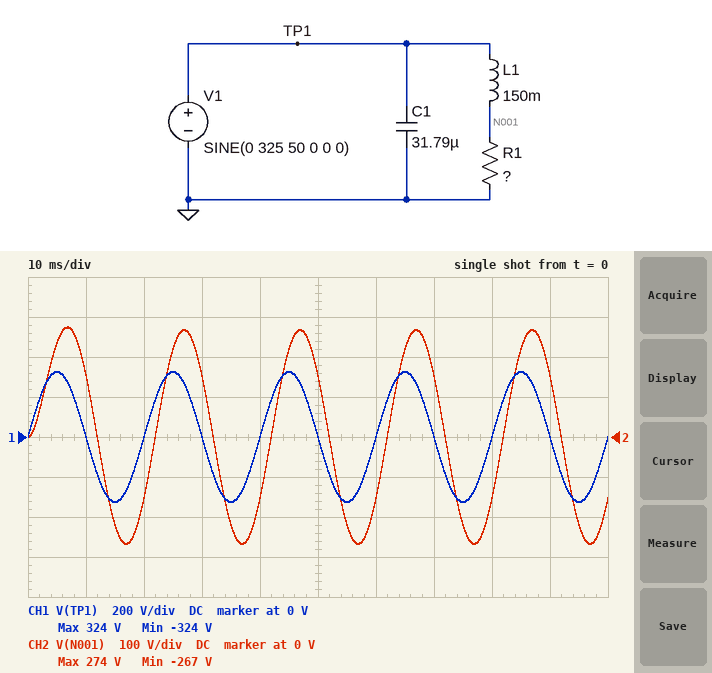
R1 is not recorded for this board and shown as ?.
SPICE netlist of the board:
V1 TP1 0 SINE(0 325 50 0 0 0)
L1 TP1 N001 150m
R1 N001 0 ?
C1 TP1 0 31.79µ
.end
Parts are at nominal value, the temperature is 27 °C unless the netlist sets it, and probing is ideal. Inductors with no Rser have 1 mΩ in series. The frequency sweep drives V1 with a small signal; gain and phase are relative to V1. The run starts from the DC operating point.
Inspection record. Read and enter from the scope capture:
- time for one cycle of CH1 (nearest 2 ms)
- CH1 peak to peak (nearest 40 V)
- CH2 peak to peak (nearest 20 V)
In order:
20 ms
640 V
540 V
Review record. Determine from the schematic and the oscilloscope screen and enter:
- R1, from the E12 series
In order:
68 Ω
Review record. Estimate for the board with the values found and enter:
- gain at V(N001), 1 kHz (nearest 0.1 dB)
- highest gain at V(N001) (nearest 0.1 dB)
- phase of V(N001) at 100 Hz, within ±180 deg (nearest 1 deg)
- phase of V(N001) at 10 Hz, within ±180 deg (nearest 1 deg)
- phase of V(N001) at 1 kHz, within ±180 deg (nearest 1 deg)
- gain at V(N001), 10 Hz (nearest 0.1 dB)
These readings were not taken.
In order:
-22.9 dB
0 dB
-54 deg
-8 deg
-86 deg
-0.1 dB
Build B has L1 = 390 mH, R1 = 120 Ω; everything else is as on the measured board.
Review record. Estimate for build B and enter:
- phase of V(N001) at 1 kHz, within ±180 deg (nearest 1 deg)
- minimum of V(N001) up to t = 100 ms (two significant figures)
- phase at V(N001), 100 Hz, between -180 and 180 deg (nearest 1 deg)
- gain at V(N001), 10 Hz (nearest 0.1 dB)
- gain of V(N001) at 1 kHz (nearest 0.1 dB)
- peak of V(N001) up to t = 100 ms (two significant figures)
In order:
-87 deg
-230 V
-64 deg
-0.2 dB
-26.2 dB
240 V
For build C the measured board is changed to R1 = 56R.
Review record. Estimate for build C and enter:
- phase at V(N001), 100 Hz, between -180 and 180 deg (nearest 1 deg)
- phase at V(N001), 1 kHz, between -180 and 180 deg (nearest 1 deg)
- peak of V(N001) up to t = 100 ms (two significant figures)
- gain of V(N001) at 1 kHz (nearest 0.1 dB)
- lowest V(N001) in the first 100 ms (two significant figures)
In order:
-59 deg
-87 deg
260 V
-24.5 dB
-250 V
